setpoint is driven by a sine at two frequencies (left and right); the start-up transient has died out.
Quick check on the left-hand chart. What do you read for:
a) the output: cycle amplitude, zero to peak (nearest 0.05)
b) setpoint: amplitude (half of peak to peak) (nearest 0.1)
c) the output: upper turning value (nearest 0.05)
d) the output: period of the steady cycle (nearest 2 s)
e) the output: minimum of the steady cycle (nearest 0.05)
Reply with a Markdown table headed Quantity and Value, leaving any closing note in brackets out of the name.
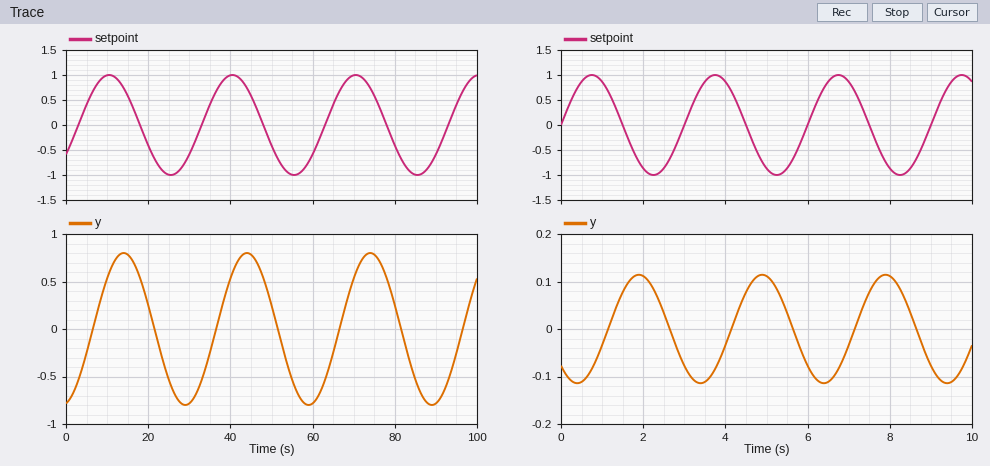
| Quantity | Value |
|---|---|
| the output: cycle amplitude, zero to peak | 0.80 |
| setpoint: amplitude (half of peak to peak) | 1.0 |
| the output: upper turning value | 0.80 |
| the output: period of the steady cycle | 30 s |
| the output: minimum of the steady cycle | -0.80 |
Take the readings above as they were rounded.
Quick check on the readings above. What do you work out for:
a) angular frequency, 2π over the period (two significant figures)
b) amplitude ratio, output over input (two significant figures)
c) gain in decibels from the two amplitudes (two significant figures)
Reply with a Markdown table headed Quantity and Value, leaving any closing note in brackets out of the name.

| Quantity | Value |
|---|---|
| angular frequency, 2π over the period | 0.21 rad/s |
| amplitude ratio, output over input | 0.80 |
| gain in decibels from the two amplitudes | -1.9 dB |
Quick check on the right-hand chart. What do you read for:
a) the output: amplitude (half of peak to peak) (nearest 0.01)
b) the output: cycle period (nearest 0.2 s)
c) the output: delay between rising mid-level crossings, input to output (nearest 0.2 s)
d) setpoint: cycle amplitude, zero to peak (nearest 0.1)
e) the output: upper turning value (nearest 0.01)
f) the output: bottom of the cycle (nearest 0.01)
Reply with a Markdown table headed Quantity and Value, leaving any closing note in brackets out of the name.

| Quantity | Value |
|---|---|
| the output: amplitude (half of peak to peak) | 0.11 |
| the output: cycle period | 3.0 s |
| the output: delay between rising mid-level crossings, input to output | 1.2 s |
| setpoint: cycle amplitude, zero to peak | 1.0 |
| the output: upper turning value | 0.11 |
| the output: bottom of the cycle | -0.11 |
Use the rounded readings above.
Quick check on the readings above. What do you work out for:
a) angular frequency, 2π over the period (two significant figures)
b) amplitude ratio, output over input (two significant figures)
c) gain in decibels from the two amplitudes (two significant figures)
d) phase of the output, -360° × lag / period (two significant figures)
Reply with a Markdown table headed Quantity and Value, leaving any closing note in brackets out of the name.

| Quantity | Value |
|---|---|
| angular frequency, 2π over the period | 2.1 rad/s |
| amplitude ratio, output over input | 0.11 |
| gain in decibels from the two amplitudes | -19 dB |
| phase of the output, -360° × lag / period | -140° |
